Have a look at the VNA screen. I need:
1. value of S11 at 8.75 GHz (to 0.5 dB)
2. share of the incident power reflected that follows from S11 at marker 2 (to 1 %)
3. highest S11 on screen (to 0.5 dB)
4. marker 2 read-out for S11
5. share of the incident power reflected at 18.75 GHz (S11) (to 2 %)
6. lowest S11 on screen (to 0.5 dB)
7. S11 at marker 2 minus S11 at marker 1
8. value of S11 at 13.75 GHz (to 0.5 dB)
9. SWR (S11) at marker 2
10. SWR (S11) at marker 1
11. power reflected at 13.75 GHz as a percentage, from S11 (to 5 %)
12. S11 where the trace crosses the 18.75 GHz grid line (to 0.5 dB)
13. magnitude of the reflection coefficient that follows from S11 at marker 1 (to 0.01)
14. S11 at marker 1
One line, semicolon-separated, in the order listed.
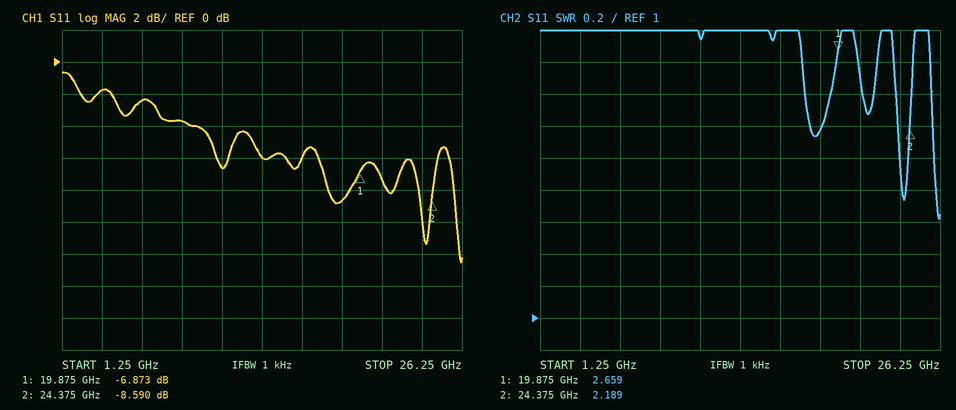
-3.5 dB; 14 %; -0.5 dB; -8.590 dB; 14 %; -12.5 dB; -1.717 dB; -6.0 dB; 2.189; 2.659; 25 %; -8.5 dB; 0.45; -6.873 dB
